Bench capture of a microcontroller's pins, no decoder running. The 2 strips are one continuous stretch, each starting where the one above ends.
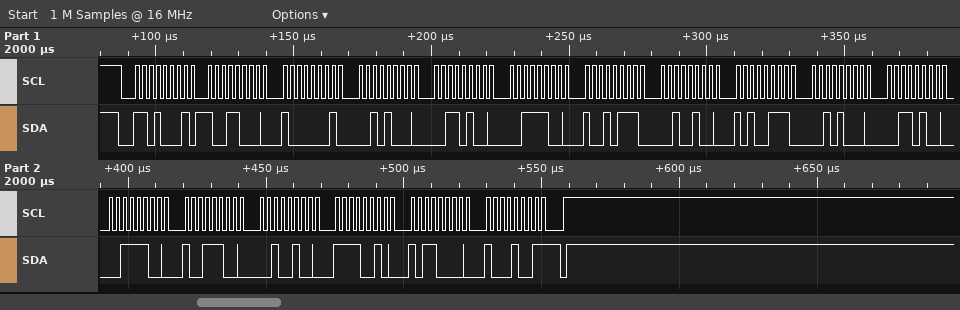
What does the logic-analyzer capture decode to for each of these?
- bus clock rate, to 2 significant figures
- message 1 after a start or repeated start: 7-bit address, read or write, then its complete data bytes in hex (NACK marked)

400 kHz
0x68 read: 98 81 28 34 3C 97 24 A7 28 34 3C 9C 24 F2 B0 89 NACK
